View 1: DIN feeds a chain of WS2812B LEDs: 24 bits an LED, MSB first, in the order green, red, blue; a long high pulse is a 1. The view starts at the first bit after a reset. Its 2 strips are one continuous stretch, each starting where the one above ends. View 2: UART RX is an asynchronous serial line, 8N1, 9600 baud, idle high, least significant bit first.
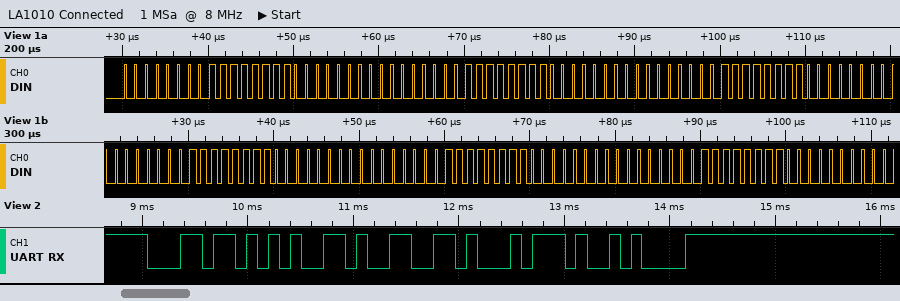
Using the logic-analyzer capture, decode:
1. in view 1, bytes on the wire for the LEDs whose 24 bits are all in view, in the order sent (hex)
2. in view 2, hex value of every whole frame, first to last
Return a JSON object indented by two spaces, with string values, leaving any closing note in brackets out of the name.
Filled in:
{
  "in view 1, bytes on the wire for the LEDs whose 24 bits are all in view, in the order sent": "00 FF 00 00 FF 00 00 FF 00 00 FF 00 00 FF 00 00 FF 00",
  "in view 2, hex value of every whole frame, first to last": "0x6C 0x65 0x66 0x74 0x0A"
}
